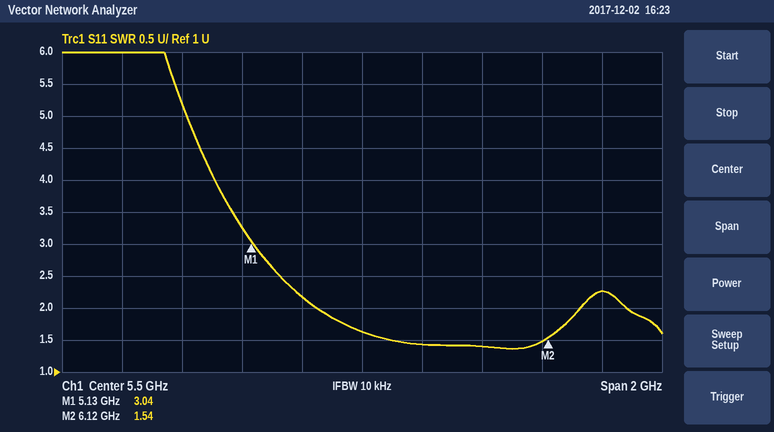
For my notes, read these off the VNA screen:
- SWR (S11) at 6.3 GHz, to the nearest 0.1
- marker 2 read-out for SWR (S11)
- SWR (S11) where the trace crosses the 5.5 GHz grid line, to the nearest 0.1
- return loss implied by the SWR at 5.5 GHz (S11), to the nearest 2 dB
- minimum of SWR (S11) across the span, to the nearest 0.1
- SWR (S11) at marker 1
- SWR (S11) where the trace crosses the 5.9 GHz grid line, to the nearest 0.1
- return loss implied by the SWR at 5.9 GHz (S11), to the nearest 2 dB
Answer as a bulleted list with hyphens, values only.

- 2.3
- 1.54
- 1.6
- 12 dB
- 1.4
- 3.04
- 1.4
- 16 dB
